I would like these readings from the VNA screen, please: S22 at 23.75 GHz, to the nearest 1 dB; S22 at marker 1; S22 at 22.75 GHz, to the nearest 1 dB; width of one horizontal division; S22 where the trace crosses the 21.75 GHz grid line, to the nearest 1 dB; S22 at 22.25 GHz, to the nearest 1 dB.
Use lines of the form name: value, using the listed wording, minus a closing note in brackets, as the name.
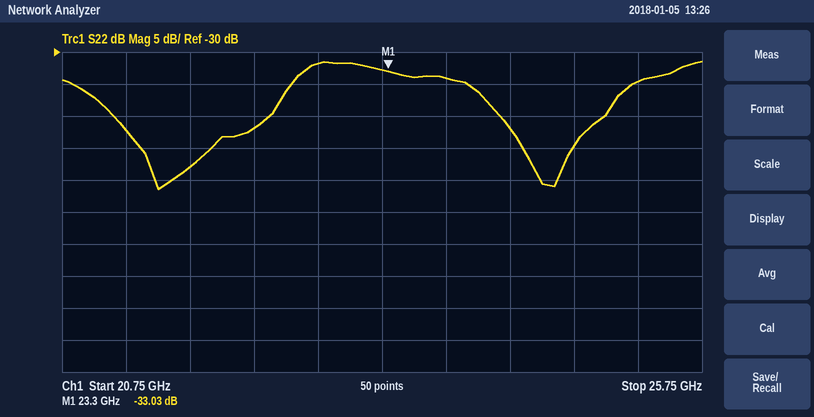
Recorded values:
S22 at 23.75 GHz, to the nearest 1 dB: -34 dB
S22 at marker 1: -33.03 dB
S22 at 22.75 GHz, to the nearest 1 dB: -32 dB
width of one horizontal division: 500 MHz
S22 where the trace crosses the 21.75 GHz grid line, to the nearest 1 dB: -48 dB
S22 at 22.25 GHz, to the nearest 1 dB: -42 dB
